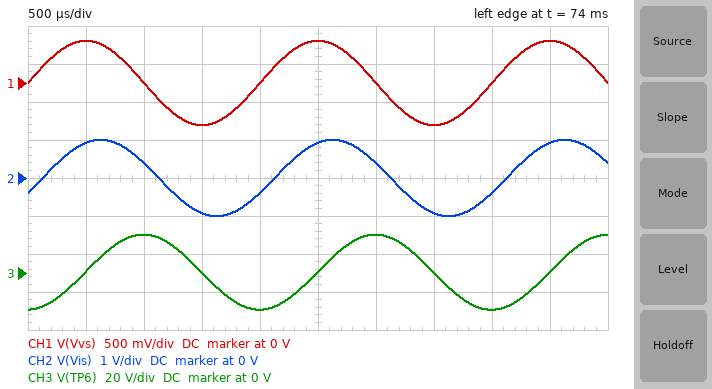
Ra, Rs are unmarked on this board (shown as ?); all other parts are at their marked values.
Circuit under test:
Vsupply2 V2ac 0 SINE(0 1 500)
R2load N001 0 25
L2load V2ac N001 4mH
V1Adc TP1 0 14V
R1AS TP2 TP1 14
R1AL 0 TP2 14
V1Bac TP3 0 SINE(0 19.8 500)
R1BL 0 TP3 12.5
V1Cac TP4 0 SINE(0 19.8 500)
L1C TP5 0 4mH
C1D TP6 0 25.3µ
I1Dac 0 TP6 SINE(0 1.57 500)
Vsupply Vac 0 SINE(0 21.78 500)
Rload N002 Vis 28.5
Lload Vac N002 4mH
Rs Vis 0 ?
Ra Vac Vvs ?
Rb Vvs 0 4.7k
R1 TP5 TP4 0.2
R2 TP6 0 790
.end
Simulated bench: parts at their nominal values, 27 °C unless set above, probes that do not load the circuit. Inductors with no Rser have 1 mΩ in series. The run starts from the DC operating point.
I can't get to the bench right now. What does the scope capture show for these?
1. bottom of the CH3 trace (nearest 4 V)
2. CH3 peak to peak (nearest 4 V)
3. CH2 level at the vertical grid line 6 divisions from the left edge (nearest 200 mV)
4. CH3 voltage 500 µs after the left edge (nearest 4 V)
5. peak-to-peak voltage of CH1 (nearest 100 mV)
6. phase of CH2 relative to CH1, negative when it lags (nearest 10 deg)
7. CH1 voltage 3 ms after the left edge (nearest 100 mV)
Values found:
-20 V
40 V
400 mV
0 V
1.1 V
-20 deg
0 V
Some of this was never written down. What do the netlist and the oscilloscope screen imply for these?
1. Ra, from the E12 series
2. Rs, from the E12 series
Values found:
180 kΩ
1.5 Ω
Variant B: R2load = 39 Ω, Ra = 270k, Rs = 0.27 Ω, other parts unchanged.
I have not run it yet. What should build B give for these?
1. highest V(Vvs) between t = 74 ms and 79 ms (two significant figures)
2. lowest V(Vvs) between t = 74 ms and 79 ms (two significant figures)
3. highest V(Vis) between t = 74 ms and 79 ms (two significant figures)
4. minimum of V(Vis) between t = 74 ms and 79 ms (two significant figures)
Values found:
370 mV
-370 mV
190 mV
-190 mV
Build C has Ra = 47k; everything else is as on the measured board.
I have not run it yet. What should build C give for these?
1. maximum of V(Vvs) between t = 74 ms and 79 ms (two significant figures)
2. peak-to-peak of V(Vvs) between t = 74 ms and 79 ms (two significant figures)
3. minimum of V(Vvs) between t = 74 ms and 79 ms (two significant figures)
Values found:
2.0 V
4.0 V
-2.0 V
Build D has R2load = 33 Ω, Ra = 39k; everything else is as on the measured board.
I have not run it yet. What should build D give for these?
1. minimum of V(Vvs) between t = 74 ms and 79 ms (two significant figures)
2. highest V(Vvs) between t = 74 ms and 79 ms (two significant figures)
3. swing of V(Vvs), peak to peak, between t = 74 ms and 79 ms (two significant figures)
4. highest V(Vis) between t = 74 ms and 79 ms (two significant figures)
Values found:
-2.3 V
2.3 V
4.7 V
1.0 V
